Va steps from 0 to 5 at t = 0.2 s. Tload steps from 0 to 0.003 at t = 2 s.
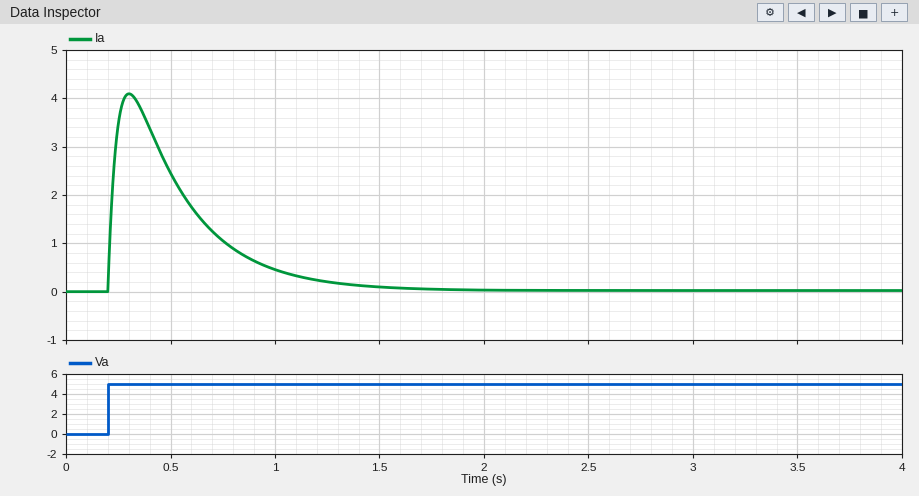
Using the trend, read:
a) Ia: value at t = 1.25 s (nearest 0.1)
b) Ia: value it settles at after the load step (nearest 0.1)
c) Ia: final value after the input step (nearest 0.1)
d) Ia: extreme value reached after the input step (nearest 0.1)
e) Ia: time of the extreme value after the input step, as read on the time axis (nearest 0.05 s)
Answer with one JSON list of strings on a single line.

["0.2", "0.0", "0.0", "4.1", "0.30 s"]
